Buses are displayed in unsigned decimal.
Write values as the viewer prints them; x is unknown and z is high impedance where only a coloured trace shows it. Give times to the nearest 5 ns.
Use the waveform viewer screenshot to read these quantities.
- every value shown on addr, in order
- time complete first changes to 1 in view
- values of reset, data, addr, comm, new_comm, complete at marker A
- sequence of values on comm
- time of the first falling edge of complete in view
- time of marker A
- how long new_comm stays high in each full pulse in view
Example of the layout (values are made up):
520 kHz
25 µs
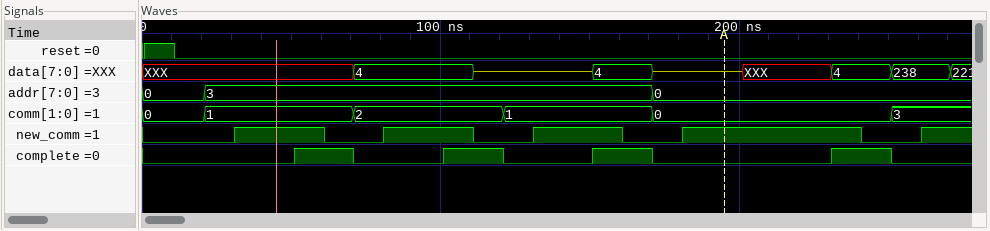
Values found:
0, 3, 0
50 ns
reset=0, data=z, addr=0, comm=0, new_comm=1, complete=0
0, 1, 2, 1, 0, 3
70 ns
195 ns
30 ns, 30 ns, 30 ns, 60 ns
